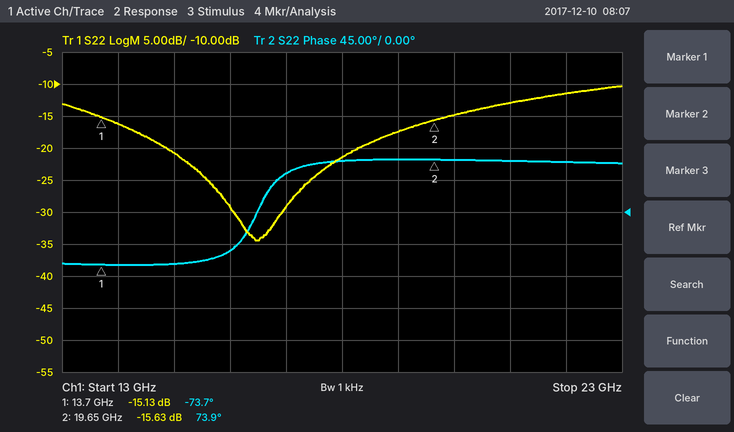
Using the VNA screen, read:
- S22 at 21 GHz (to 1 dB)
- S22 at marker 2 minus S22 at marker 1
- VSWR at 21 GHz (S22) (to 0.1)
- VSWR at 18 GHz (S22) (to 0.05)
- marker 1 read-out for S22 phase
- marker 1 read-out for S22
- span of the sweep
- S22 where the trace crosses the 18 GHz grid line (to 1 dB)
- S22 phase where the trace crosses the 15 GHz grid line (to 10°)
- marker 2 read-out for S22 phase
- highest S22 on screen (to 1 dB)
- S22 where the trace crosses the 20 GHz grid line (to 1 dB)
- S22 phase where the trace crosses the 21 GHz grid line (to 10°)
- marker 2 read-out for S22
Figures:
-13 dB
-0.50 dB
1.6
1.20
-73.7°
-15.13 dB
10 GHz
-21 dB
-70°
73.9°
-10 dB
-15 dB
70°
-15.63 dB
